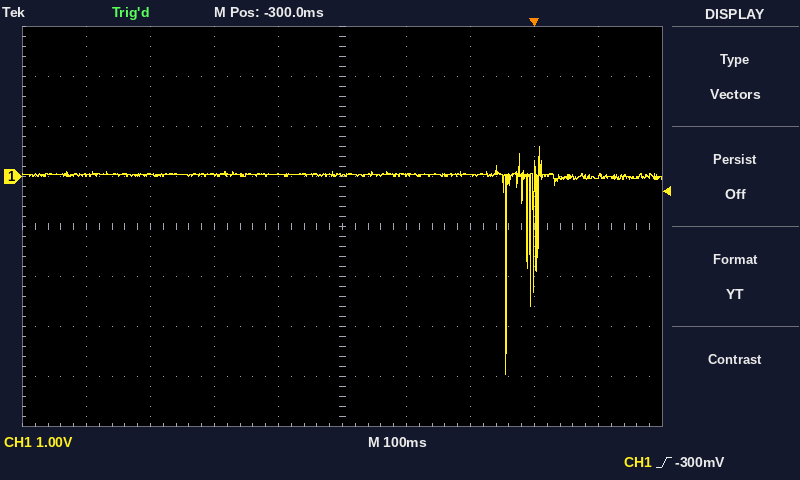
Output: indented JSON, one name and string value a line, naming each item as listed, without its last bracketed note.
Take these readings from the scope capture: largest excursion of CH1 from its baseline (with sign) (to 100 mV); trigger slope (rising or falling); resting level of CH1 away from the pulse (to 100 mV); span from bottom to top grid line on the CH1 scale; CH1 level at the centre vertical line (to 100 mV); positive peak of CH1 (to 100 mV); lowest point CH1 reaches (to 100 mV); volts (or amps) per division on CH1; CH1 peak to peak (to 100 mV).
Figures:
{
  "largest excursion of CH1 from its baseline (with sign)": "-4.0 V",
  "trigger slope": "rising",
  "resting level of CH1 away from the pulse": "0.0 V",
  "span from bottom to top grid line on the CH1 scale": "8 V",
  "CH1 level at the centre vertical line": "0.0 V",
  "positive peak of CH1": "600 mV",
  "lowest point CH1 reaches": "-4.0 V",
  "volts (or amps) per division on CH1": "1 V",
  "CH1 peak to peak": "4.6 V"
}
